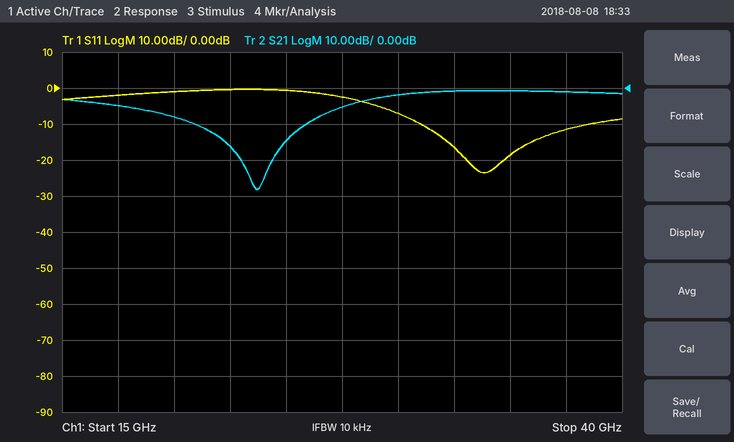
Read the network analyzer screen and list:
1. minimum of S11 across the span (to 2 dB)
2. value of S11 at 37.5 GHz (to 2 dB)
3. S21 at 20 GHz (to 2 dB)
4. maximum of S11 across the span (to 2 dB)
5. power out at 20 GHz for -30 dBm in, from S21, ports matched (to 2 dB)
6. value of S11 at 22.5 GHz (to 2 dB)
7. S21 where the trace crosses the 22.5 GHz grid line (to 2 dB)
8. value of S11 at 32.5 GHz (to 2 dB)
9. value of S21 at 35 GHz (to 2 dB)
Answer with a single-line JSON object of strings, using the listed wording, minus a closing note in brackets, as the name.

{"minimum of S11 across the span": "-24 dB", "value of S11 at 37.5 GHz": "-12 dB", "S21 at 20 GHz": "-8 dB", "maximum of S11 across the span": "0 dB", "power out at 20 GHz for -30 dBm in, from S21, ports matched": "-38 dBm", "value of S11 at 22.5 GHz": "0 dB", "S21 where the trace crosses the 22.5 GHz grid line": "-16 dB", "value of S11 at 32.5 GHz": "-16 dB", "value of S21 at 35 GHz": "0 dB"}
